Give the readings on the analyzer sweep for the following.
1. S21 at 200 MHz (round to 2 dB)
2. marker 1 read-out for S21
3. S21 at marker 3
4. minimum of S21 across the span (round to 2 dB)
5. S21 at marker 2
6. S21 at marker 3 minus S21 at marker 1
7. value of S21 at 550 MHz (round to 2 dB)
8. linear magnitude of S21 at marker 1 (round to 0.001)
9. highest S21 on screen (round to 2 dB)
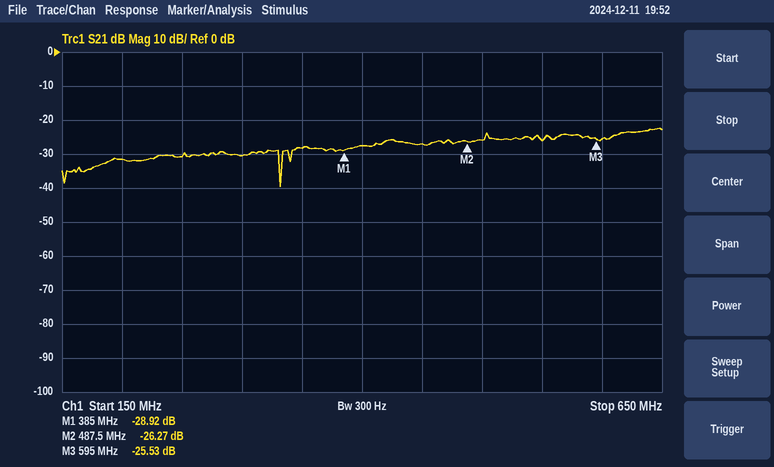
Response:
-32 dB
-28.92 dB
-25.53 dB
-40 dB
-26.27 dB
3.39 dB
-26 dB
0.036
-22 dB
